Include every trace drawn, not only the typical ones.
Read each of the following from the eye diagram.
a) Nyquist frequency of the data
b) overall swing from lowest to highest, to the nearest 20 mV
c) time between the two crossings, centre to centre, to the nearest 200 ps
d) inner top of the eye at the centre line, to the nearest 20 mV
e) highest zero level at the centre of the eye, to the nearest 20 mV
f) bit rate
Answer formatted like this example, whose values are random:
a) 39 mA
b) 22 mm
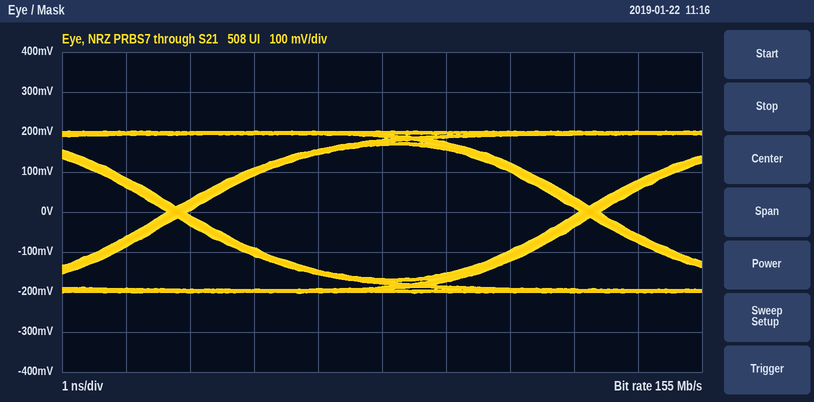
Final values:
a) 77.5 MHz
b) 400 mV
c) 6.4 ns
d) 160 mV
e) -160 mV
f) 155 Mb/s
